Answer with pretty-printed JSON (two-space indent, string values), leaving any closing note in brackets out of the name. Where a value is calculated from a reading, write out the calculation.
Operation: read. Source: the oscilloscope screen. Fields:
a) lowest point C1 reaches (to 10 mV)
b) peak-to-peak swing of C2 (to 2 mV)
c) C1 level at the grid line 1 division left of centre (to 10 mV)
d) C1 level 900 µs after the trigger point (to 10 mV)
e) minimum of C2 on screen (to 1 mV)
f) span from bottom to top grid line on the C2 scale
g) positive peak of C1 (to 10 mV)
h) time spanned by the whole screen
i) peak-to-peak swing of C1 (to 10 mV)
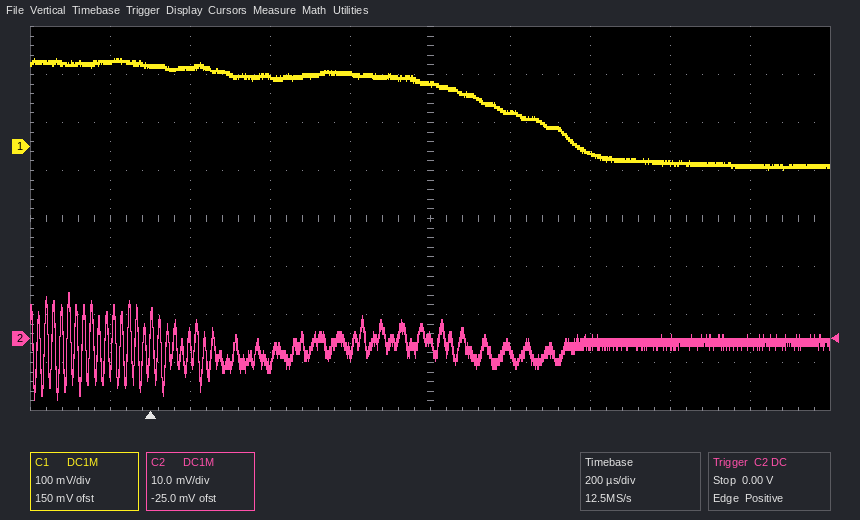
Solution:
{
  "lowest point C1 reaches": "-50 mV",
  "peak-to-peak swing of C2": "22 mV",
  "C1 level at the grid line 1 division left of centre": "150 mV",
  "C1 level 900 µs after the trigger point": "70 mV",
  "minimum of C2 on screen": "-13 mV",
  "span from bottom to top grid line on the C2 scale": "80 mV",
  "positive peak of C1": "180 mV",
  "time spanned by the whole screen": "2 ms",
  "peak-to-peak swing of C1": "180 mV − (-50 mV) = 230 mV"
}
